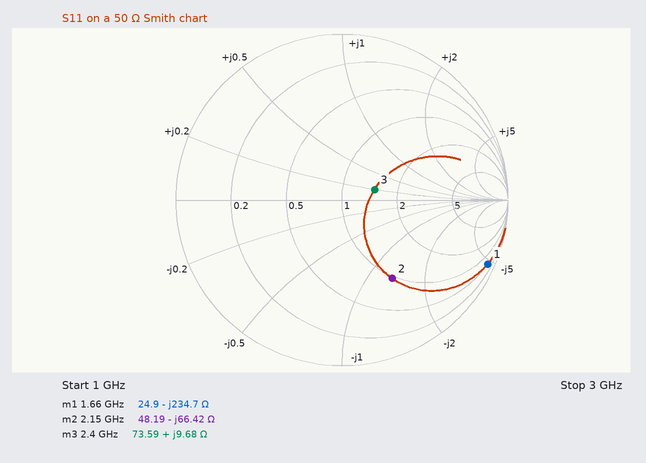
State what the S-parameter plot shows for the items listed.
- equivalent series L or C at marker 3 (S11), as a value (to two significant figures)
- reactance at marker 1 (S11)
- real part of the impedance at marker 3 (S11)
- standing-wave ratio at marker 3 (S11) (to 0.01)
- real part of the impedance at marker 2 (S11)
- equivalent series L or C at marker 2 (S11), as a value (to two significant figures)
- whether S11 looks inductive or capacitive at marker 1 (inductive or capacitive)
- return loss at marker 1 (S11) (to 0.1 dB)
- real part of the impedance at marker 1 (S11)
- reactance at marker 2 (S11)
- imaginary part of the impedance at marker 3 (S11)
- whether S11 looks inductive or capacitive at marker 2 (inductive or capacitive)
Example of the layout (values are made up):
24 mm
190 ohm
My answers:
640 pH
-234.7 Ω
73.59 Ω
1.52
48.19 Ω
1.1 pF
capacitive
0.4 dB
24.9 Ω
-66.42 Ω
+9.68 Ω
capacitive
